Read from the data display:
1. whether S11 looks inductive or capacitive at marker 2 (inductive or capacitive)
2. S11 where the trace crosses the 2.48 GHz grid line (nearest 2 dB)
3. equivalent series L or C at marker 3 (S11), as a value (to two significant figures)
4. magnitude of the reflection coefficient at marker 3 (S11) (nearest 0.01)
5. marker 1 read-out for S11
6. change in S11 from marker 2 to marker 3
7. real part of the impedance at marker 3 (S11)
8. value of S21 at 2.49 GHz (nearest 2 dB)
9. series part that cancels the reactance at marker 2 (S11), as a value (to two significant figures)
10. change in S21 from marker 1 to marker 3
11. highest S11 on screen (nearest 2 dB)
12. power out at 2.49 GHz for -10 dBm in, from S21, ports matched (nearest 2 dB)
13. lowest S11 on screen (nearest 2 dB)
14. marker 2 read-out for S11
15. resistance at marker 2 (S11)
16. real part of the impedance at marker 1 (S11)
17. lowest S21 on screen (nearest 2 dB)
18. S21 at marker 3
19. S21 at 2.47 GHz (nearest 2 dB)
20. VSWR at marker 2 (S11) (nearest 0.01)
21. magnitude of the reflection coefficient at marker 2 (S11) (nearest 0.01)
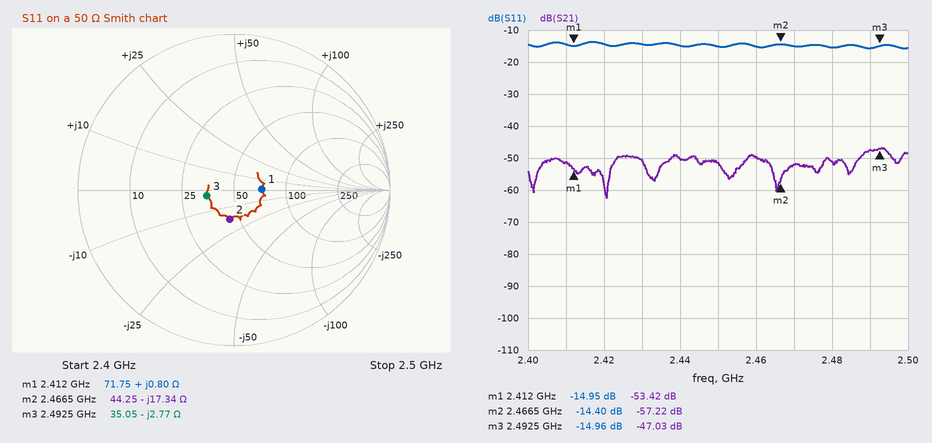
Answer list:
capacitive
-16 dB
23 pF
0.18
-14.95 dB
-0.56 dB
35.05 Ω
-48 dB
1.1 nH
6.39 dB
-14 dB
-58 dBm
-16 dB
-14.40 dB
44.25 Ω
71.75 Ω
-62 dB
-47.03 dB
-52 dB
1.47
0.19
